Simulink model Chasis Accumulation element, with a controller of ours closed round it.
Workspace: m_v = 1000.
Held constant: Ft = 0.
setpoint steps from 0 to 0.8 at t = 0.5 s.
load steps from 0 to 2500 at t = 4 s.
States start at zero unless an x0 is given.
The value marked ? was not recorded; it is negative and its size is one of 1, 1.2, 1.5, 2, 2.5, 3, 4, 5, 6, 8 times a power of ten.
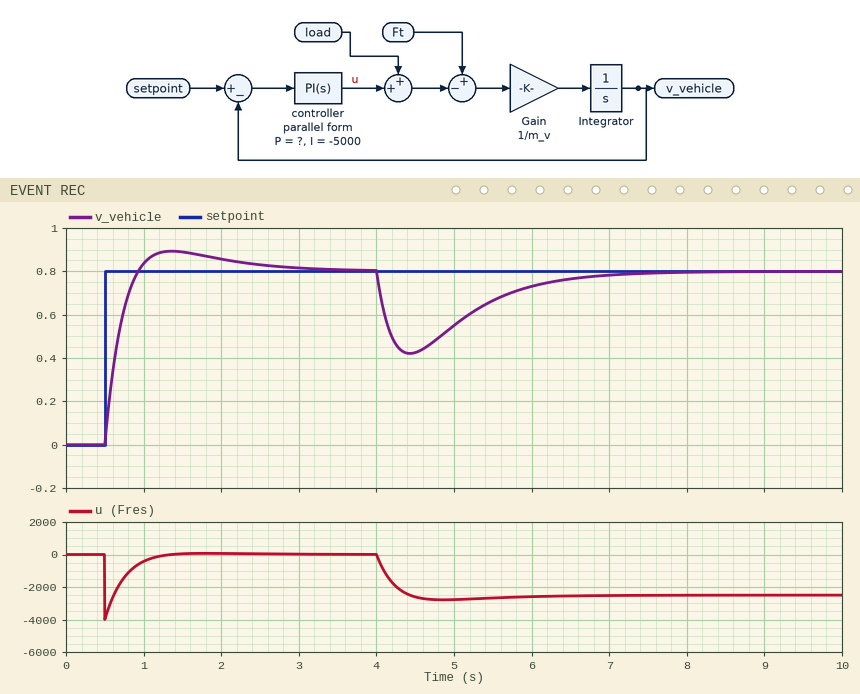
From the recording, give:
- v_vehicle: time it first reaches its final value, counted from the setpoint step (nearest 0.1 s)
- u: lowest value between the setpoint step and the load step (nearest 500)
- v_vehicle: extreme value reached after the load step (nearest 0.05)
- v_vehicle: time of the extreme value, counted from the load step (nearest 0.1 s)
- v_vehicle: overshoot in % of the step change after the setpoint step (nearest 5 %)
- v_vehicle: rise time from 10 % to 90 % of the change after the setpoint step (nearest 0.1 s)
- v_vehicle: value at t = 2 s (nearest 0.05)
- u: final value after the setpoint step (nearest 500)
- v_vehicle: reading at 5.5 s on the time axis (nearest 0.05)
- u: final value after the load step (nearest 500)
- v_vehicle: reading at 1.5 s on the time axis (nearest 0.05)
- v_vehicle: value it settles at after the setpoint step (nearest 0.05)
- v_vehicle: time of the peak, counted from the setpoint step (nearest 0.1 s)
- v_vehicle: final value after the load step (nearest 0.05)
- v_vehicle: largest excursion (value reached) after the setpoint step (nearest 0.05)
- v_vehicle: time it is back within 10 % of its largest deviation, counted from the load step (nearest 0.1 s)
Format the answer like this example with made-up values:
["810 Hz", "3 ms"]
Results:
["0.4 s", "-4000", "0.40", "0.4 s", "10 %", "0.3 s", "0.85", "0", "0.65", "-2500", "0.90", "0.80", "0.9 s", "0.80", "0.90", "2.4 s"]
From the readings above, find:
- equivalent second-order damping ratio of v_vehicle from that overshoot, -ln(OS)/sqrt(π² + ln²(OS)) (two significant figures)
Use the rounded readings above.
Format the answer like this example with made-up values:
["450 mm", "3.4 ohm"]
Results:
["0.59"]
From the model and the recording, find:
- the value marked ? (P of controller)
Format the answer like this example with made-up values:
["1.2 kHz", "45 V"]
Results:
["-5000"]
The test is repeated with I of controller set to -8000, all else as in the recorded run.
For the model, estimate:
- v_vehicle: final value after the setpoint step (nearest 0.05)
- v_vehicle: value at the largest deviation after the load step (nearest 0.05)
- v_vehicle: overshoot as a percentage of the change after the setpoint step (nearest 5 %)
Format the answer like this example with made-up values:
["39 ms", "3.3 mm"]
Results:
["0.80", "0.45", "15 %"]
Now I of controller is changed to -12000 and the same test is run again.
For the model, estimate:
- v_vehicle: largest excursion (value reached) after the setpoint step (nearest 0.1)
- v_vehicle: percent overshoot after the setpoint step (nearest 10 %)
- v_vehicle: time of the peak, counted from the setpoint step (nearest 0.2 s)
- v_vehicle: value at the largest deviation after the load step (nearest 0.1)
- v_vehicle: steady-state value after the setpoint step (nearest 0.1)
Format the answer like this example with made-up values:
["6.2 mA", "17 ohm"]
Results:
["1.0", "20 %", "0.6 s", "0.5", "0.8"]
